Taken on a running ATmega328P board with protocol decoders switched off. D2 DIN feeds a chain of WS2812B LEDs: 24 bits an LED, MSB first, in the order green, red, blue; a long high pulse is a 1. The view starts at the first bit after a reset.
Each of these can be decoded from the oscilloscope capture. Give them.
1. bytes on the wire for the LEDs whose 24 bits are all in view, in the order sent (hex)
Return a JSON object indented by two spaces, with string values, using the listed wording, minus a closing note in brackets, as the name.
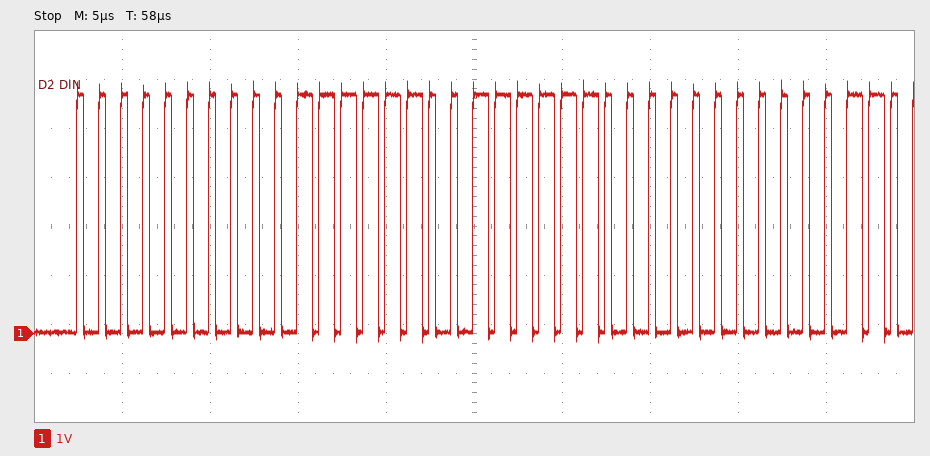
{
  "bytes on the wire for the LEDs whose 24 bits are all in view, in the order sent": "00 3F 3F"
}
